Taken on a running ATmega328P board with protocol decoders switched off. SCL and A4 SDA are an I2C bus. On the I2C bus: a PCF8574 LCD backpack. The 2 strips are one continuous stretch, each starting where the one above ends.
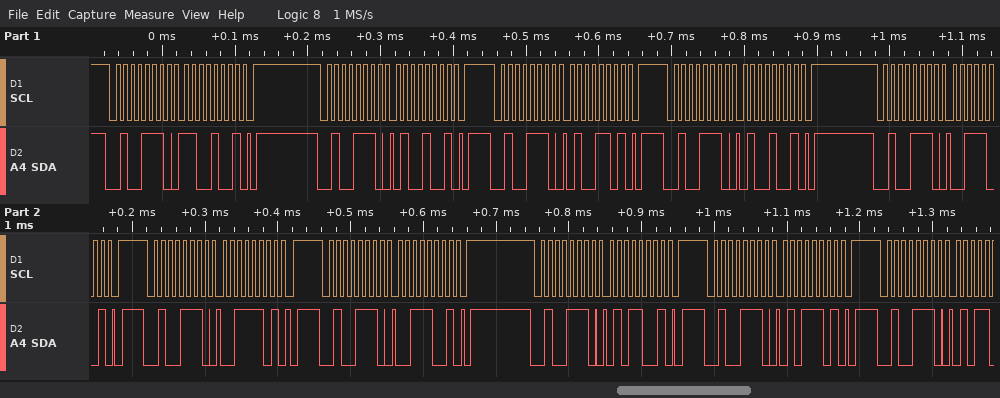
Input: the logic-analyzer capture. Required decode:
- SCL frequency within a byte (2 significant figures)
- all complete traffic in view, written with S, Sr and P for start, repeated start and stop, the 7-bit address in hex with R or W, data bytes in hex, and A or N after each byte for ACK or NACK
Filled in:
100 kHz
S 27W A C9 A P S 27W A 49 A P S 27W A 4D A P S 27W A 49 A P S 27W A 39 A P S 27W A 3D A P S 27W A 39 A P S 27W A 59 A P S 27W A 5D A P S 27W A
